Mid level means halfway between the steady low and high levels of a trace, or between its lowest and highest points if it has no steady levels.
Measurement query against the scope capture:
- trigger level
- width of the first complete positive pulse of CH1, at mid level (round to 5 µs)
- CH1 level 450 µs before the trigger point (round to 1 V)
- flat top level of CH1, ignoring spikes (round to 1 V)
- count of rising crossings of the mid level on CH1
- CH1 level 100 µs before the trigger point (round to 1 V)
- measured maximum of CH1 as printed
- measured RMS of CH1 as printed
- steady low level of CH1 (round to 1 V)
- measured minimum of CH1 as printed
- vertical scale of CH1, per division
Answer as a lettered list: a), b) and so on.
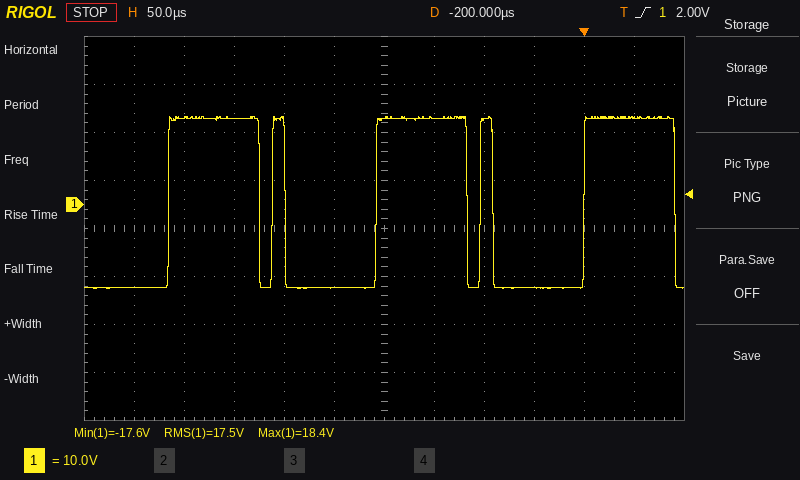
a) 2.00 V
b) 90 µs
c) -17 V
d) 18 V
e) 5
f) 18 V
g) 18.4 V
h) 17.5 V
i) -17 V
j) -17.6 V
k) 10 V
